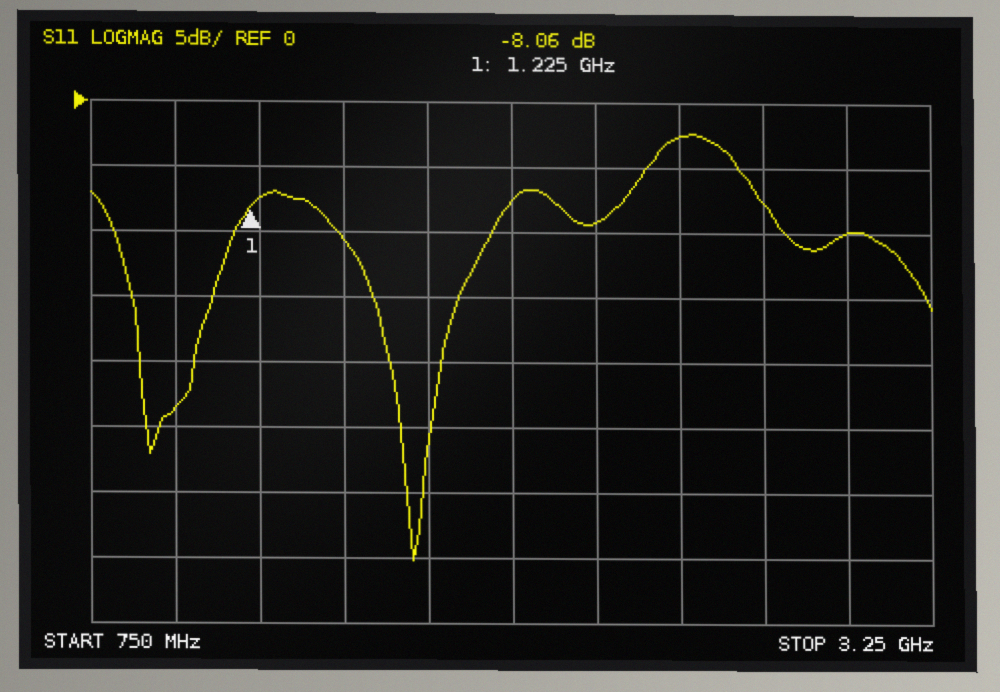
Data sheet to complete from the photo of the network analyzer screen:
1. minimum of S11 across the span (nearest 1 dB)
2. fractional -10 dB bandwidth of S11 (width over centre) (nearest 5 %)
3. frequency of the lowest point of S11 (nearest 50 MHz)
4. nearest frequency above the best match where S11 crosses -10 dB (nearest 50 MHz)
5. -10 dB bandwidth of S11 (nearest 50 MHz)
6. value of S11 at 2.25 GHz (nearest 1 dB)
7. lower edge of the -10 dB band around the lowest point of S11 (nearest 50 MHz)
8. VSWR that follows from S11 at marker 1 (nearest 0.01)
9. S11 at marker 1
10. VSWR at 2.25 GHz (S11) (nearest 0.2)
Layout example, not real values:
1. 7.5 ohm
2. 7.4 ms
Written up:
1. -35 dB
2. 25 %
3. 1.70 GHz
4. 1.95 GHz
5. 450 MHz
6. -9 dB
7. 1.50 GHz
8. 2.31
9. -8.06 dB
10. 2.0
